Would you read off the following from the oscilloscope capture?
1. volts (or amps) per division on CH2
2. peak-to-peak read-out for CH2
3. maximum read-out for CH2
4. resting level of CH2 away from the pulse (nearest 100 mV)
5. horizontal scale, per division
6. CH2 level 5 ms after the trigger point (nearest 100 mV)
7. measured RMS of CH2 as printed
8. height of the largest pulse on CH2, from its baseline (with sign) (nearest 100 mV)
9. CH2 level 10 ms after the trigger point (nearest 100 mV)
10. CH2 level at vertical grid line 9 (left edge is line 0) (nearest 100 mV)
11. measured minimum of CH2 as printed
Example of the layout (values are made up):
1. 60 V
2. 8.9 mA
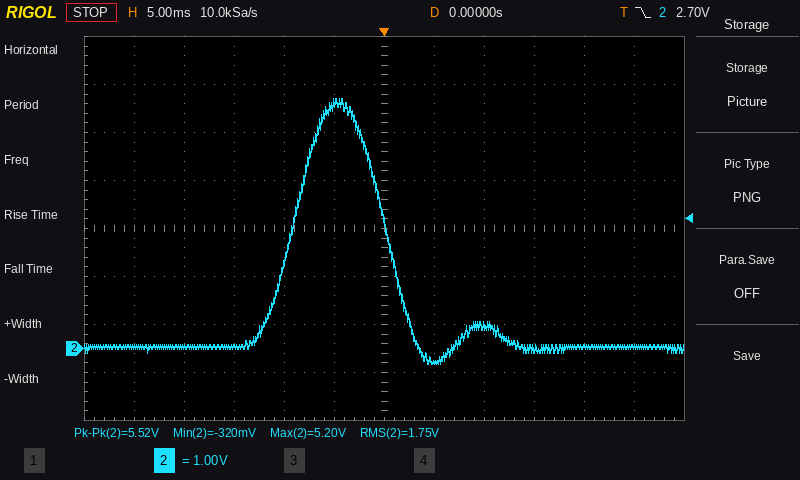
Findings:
1. 1 V
2. 5.52 V
3. 5.20 V
4. 0.0 V
5. 5 ms
6. -300 mV
7. 1.75 V
8. +5.2 V
9. 500 mV
10. 0.0 V
11. -320 mV
